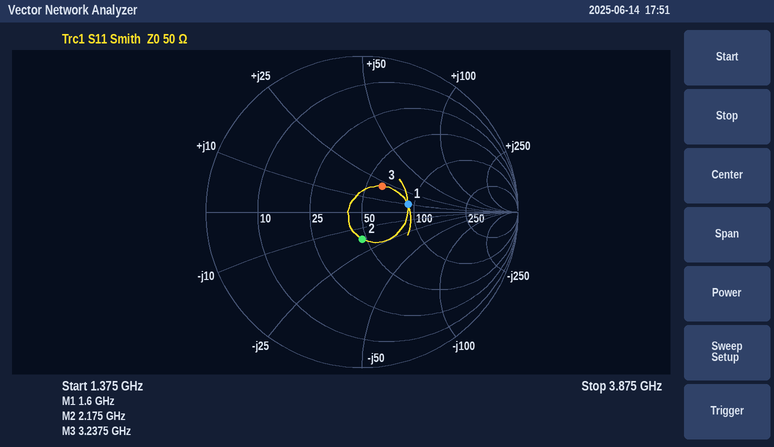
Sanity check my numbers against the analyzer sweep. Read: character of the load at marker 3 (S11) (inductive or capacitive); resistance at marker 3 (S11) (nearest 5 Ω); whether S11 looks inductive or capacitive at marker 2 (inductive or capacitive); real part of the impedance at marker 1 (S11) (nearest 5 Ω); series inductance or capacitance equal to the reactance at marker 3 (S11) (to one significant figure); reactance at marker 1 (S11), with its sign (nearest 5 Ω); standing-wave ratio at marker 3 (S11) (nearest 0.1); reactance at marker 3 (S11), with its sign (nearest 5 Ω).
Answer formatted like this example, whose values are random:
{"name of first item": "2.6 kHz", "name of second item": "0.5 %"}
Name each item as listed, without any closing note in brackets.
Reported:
{"character of the load at marker 3 (S11)": "inductive", "resistance at marker 3 (S11)": "60 Ω", "whether S11 looks inductive or capacitive at marker 2": "capacitive", "real part of the impedance at marker 1 (S11)": "90 Ω", "series inductance or capacitance equal to the reactance at marker 3 (S11)": "1 nH", "reactance at marker 1 (S11), with its sign": "+10 Ω", "standing-wave ratio at marker 3 (S11)": "1.5", "reactance at marker 3 (S11), with its sign": "+20 Ω"}
